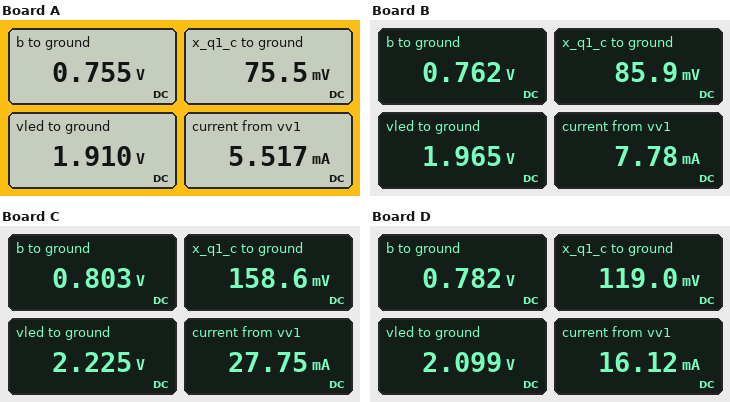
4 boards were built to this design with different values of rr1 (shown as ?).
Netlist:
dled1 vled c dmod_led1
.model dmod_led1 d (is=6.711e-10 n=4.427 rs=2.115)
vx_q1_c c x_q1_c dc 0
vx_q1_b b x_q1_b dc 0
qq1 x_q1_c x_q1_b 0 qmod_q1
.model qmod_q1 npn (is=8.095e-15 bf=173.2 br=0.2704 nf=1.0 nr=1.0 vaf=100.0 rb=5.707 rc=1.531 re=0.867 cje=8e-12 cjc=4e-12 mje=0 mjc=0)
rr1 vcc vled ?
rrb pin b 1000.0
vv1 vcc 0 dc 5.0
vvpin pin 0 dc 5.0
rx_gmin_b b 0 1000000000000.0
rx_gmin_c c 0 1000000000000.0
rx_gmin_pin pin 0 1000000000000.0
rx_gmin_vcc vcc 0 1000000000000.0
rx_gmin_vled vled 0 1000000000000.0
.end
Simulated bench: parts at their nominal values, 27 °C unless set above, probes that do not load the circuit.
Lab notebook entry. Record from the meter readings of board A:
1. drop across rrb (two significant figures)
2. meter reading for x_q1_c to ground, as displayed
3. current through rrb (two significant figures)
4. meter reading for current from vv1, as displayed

4.2 V
75.5 mV
4.2 mA
5.517 mA
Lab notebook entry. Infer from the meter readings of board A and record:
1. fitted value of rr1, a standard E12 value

560 Ω
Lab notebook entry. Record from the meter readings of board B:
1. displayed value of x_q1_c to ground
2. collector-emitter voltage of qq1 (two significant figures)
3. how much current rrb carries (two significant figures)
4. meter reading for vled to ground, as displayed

85.9 mV
86 mV
4.2 mA
1.965 V
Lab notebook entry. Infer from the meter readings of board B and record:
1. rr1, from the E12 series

390 Ω
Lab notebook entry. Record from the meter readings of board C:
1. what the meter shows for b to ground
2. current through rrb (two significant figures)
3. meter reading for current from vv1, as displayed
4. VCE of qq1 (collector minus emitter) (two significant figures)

0.803 V
4.2 mA
27.75 mA
160 mV
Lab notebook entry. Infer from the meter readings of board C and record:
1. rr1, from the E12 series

100 Ω
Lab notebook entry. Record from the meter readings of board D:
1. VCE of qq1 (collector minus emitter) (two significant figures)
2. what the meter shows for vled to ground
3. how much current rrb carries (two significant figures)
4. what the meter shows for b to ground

120 mV
2.099 V
4.2 mA
0.782 V
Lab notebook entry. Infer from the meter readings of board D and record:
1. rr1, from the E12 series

180 Ω
